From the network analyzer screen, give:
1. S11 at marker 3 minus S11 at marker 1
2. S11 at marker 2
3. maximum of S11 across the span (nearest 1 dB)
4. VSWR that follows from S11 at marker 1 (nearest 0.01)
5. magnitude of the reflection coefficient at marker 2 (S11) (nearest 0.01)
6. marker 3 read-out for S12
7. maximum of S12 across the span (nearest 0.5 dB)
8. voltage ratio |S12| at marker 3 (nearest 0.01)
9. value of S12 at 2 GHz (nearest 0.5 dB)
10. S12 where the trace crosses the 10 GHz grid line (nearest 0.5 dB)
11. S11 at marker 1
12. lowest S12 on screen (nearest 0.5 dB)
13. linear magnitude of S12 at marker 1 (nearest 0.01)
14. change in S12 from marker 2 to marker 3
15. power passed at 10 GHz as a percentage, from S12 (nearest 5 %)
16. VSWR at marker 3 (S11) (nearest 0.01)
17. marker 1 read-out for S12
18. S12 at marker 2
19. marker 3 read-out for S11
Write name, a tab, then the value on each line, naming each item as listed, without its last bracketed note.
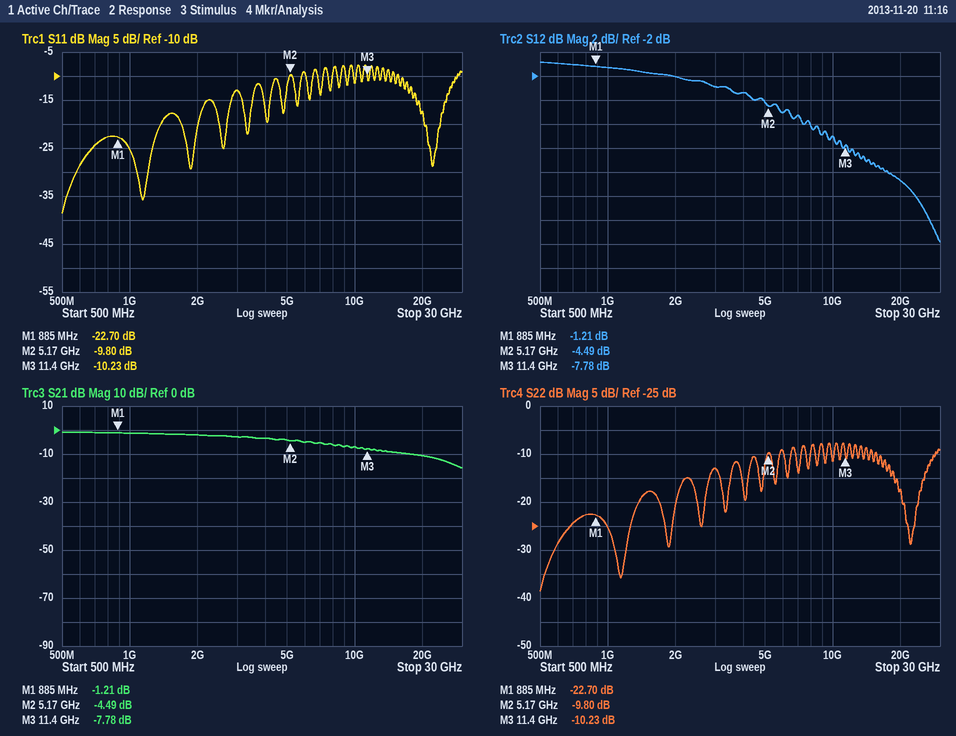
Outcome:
S11 at marker 3 minus S11 at marker 1	12.47 dB
S11 at marker 2	-9.80 dB
maximum of S11 across the span	-8 dB
VSWR that follows from S11 at marker 1	1.16
magnitude of the reflection coefficient at marker 2 (S11)	0.32
marker 3 read-out for S12	-7.78 dB
maximum of S12 across the span	-1.0 dB
voltage ratio |S12| at marker 3	0.41
value of S12 at 2 GHz	-2.0 dB
S12 where the trace crosses the 10 GHz grid line	-7.0 dB
S11 at marker 1	-22.70 dB
lowest S12 on screen	-16.0 dB
linear magnitude of S12 at marker 1	0.87
change in S12 from marker 2 to marker 3	-3.29 dB
power passed at 10 GHz as a percentage, from S12	20 %
VSWR at marker 3 (S11)	1.89
marker 1 read-out for S12	-1.21 dB
S12 at marker 2	-4.49 dB
marker 3 read-out for S11	-10.23 dB
